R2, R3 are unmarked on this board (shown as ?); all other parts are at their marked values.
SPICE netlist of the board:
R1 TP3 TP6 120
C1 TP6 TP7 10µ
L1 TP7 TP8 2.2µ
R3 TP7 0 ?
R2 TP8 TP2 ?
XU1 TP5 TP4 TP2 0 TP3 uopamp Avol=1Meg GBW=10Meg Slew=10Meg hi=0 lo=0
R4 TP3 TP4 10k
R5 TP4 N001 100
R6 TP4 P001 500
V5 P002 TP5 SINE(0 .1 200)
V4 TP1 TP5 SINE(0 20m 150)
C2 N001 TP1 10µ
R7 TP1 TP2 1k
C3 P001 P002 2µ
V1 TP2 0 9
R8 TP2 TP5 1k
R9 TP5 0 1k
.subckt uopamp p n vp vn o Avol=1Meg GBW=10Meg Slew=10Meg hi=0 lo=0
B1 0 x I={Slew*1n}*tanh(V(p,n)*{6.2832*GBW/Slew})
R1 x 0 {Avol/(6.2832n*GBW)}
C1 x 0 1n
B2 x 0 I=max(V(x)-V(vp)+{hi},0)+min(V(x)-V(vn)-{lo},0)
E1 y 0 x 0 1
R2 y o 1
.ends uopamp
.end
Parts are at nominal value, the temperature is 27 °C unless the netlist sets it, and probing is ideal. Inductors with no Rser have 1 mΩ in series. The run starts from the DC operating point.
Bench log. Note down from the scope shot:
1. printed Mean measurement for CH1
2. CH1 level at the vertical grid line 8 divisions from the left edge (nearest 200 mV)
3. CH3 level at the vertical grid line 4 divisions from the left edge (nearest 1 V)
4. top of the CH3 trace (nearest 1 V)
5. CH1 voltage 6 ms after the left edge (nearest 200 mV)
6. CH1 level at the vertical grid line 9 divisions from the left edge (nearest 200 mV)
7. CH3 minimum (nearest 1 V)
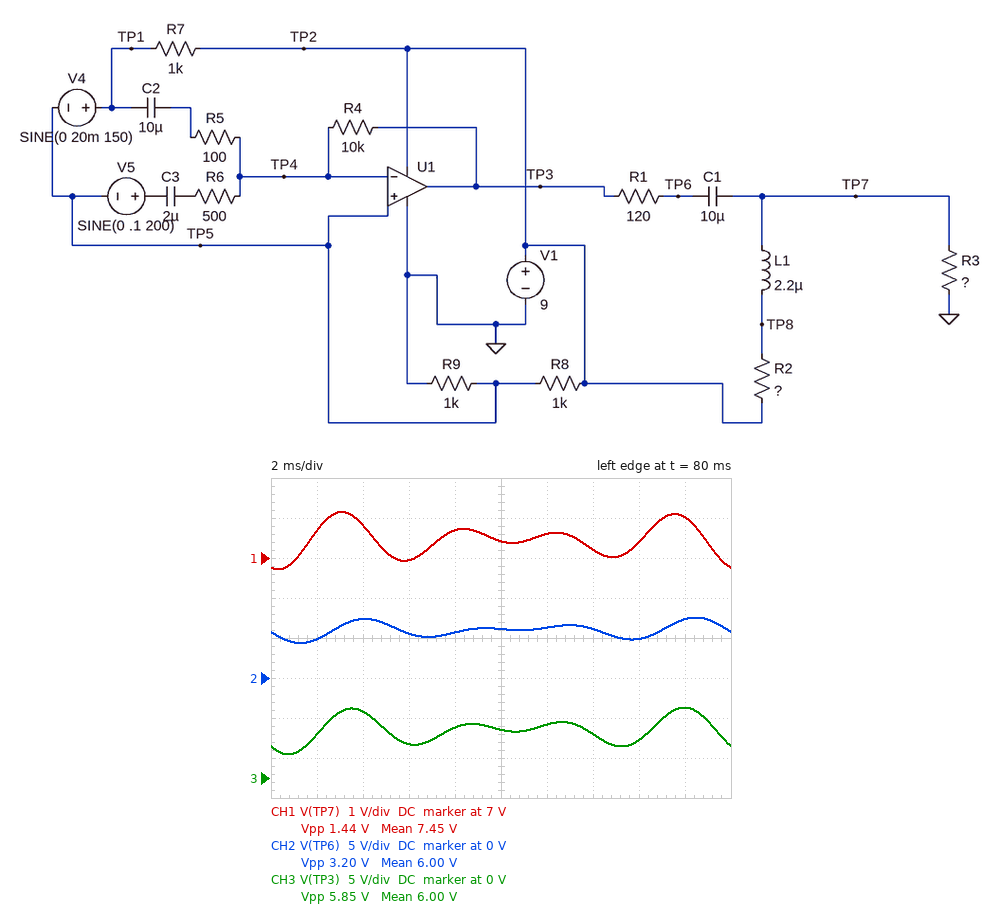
7.45 V
7.4 V
6 V
9 V
7.0 V
8.0 V
3 V
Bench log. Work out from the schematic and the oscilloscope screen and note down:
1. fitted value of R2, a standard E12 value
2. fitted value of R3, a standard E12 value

56 Ω
270 Ω
